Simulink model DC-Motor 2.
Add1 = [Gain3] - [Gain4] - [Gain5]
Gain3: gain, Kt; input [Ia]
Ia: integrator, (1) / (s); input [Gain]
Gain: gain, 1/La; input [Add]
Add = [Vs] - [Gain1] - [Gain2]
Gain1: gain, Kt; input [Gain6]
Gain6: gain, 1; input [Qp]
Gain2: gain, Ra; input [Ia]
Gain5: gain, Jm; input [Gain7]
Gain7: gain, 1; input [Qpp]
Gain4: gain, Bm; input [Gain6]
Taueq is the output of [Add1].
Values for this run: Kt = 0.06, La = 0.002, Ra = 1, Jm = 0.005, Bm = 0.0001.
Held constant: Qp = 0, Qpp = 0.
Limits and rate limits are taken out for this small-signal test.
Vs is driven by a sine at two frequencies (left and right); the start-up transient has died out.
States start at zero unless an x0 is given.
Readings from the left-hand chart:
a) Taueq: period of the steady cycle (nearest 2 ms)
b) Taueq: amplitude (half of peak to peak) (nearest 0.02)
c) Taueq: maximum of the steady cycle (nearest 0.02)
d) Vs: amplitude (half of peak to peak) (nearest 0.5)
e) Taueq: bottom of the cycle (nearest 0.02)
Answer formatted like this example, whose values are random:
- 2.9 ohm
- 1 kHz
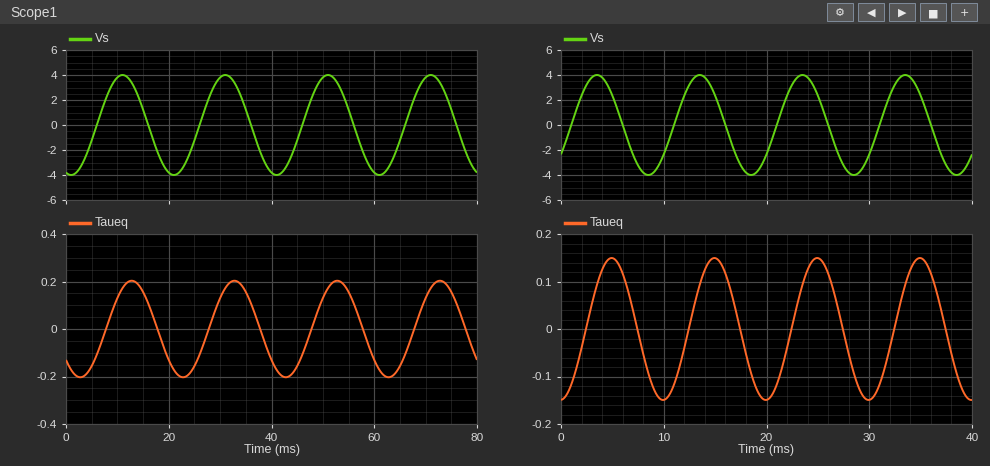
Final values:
- 20 ms
- 0.20
- 0.20
- 4.0
- -0.20
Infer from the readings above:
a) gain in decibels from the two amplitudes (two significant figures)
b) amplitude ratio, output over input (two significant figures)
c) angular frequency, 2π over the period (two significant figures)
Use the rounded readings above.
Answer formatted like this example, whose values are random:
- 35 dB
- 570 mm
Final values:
- -26 dB
- 0.050
- 0.31 rad/ms
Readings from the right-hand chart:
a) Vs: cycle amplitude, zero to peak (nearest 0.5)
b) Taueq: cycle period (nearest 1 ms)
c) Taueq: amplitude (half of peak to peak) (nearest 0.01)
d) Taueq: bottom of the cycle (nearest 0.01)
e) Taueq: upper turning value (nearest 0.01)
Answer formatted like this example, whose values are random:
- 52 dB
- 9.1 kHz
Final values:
- 4.0
- 10 ms
- 0.15
- -0.15
- 0.15
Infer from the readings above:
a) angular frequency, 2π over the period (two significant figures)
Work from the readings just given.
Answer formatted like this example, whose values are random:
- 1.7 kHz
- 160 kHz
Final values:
- 0.63 rad/ms
